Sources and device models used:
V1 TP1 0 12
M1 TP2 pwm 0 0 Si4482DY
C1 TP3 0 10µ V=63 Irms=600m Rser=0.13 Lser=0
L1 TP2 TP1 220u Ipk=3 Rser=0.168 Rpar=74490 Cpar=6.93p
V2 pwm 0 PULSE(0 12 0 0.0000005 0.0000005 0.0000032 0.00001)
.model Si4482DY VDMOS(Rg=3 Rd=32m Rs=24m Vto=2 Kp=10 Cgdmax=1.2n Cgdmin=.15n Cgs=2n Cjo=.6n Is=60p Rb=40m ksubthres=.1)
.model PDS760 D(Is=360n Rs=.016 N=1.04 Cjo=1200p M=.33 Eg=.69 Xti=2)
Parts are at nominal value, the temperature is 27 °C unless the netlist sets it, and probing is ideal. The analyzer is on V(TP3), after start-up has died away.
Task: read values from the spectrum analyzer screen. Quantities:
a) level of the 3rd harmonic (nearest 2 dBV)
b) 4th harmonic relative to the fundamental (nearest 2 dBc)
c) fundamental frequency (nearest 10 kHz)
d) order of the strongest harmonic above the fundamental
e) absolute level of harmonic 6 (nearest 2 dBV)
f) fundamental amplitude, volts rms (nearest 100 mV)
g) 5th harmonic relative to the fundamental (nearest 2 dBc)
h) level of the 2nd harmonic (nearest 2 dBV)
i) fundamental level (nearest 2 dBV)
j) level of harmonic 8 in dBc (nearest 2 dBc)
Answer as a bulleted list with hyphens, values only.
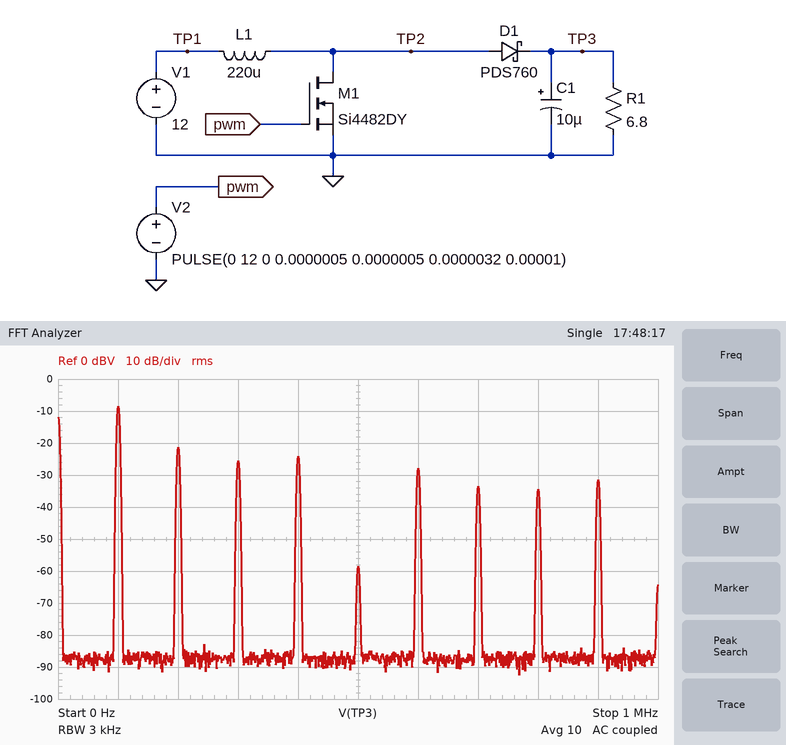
- -26 dBV
- -16 dBc
- 100 kHz
- 2
- -28 dBV
- 400 mV
- -50 dBc
- -22 dBV
- -8 dBV
- -26 dBc
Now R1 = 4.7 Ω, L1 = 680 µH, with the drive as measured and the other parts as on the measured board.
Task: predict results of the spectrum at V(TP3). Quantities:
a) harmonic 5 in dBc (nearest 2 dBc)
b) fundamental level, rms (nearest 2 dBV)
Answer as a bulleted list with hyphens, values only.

- -52 dBc
- -6 dBV
